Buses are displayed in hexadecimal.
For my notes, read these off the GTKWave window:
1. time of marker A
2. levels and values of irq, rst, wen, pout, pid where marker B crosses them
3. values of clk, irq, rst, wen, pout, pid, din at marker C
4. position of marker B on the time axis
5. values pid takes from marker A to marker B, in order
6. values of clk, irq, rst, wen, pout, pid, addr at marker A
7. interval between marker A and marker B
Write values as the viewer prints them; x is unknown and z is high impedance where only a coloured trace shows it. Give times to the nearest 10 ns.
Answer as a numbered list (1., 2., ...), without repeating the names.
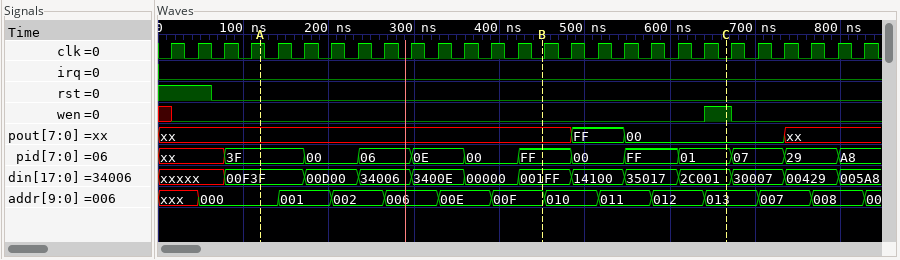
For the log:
1. 120 ns
2. irq=0, rst=0, wen=0, pout=xx, pid=FF
3. clk=0, irq=0, rst=0, wen=1, pout=00, pid=01, din=2C001
4. 450 ns
5. 3F, 00, 06, 0E, 00, FF
6. clk=1, irq=0, rst=0, wen=0, pout=xx, pid=3F, addr=000
7. 330 ns
